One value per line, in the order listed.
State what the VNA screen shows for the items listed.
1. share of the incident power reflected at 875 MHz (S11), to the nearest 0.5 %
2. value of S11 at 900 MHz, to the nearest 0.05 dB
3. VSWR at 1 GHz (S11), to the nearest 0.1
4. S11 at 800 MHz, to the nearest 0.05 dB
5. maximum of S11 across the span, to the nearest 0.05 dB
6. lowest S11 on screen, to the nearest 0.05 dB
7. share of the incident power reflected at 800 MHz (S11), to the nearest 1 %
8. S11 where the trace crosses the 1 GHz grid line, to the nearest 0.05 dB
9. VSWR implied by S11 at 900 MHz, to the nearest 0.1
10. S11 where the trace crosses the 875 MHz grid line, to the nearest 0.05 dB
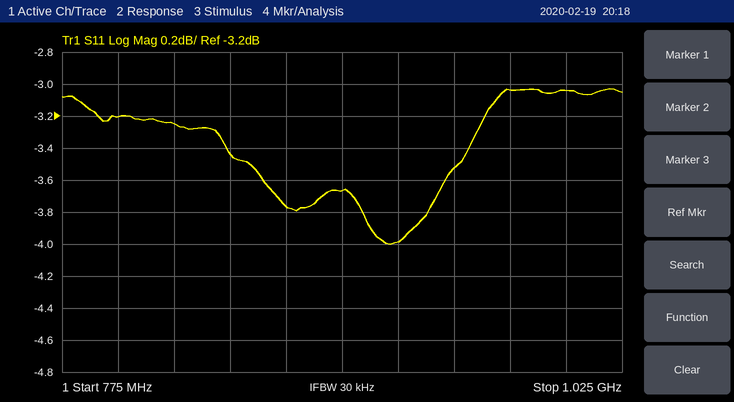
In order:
42.0 %
-3.65 dB
5.8
-3.20 dB
-3.05 dB
-4.00 dB
48 %
-3.05 dB
4.8
-3.75 dB
